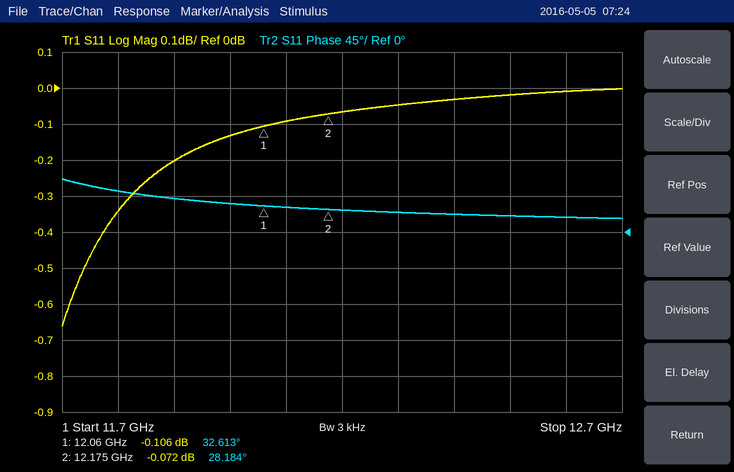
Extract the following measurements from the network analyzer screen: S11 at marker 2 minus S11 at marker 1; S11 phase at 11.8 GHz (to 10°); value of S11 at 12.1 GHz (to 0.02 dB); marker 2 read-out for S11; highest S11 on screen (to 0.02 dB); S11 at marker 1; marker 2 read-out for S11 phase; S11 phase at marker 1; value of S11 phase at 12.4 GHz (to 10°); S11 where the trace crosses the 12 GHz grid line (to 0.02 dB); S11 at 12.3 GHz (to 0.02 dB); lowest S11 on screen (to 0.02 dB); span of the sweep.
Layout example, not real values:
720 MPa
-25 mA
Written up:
0.034 dB
50°
-0.10 dB
-0.072 dB
0.00 dB
-0.106 dB
28.184°
32.613°
20°
-0.14 dB
-0.04 dB
-0.66 dB
1 GHz
